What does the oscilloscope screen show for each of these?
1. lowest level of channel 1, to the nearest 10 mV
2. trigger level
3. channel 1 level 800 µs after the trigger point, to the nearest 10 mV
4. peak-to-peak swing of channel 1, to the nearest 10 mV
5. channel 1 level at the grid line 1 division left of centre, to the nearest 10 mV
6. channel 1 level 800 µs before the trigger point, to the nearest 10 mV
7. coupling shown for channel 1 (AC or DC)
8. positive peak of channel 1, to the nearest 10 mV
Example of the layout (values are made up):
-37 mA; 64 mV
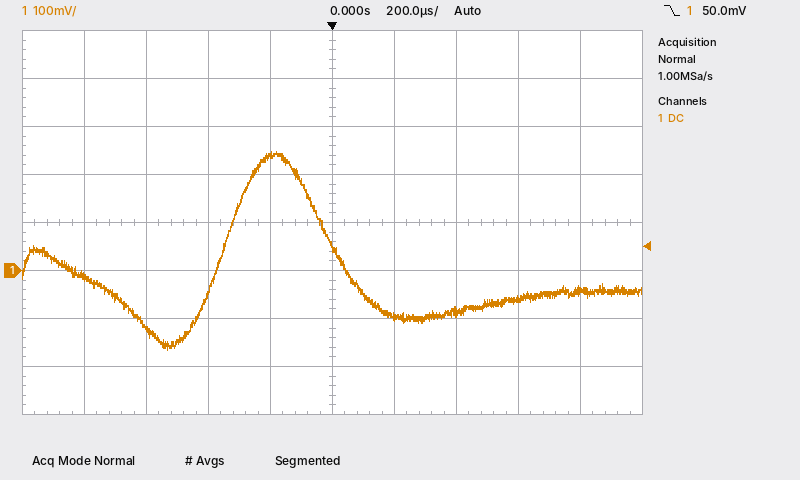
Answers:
-160 mV; 50.0 mV; -40 mV; 410 mV; 240 mV; -10 mV; DC; 250 mV
